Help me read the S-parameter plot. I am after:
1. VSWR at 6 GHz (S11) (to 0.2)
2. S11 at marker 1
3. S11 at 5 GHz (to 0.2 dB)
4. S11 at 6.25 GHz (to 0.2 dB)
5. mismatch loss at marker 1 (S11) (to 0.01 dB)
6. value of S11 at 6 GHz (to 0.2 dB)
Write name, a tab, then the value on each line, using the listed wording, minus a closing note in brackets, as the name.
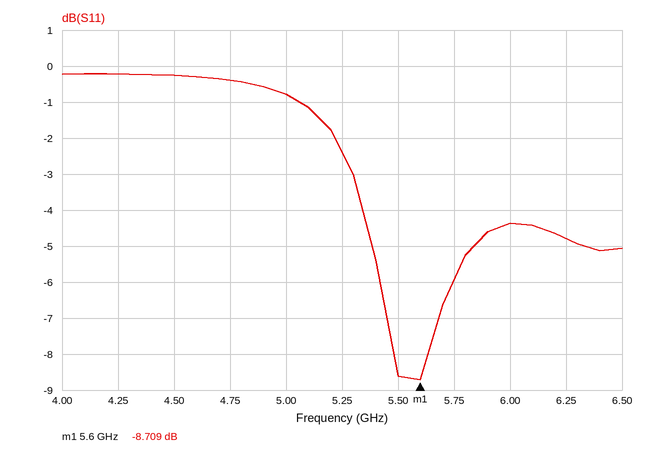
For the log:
VSWR at 6 GHz (S11)	4.0
S11 at marker 1	-8.709 dB
S11 at 5 GHz	-0.8 dB
S11 at 6.25 GHz	-4.8 dB
mismatch loss at marker 1 (S11)	0.63 dB
value of S11 at 6 GHz	-4.4 dB
